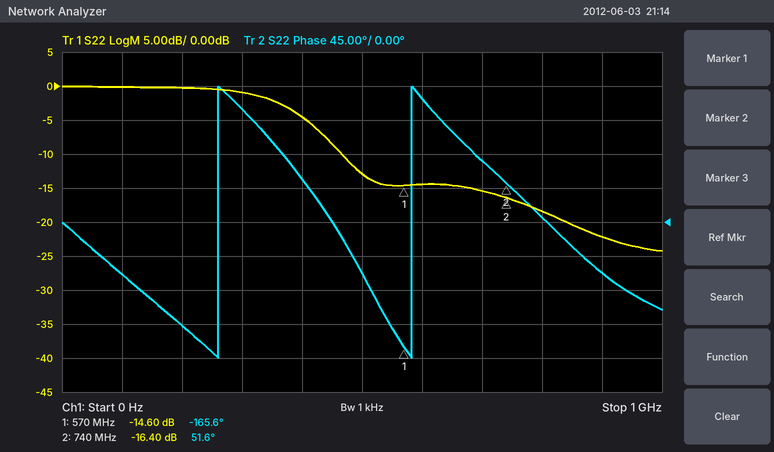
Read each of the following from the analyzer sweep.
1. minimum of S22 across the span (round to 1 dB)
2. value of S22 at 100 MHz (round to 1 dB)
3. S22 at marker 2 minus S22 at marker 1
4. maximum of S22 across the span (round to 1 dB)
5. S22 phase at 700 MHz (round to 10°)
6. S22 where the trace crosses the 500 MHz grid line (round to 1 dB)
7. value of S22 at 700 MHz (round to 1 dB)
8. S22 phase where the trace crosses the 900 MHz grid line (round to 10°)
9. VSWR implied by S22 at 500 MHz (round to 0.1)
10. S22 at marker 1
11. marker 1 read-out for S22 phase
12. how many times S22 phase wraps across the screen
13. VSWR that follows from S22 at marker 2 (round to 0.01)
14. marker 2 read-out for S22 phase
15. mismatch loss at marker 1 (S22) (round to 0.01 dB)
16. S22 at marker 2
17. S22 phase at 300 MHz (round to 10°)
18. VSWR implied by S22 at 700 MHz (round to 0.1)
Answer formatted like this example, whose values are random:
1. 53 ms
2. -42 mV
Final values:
1. -24 dB
2. 0 dB
3. -1.80 dB
4. 0 dB
5. 80°
6. -13 dB
7. -15 dB
8. -70°
9. 1.6
10. -14.60 dB
11. -165.6°
12. 2
13. 1.36
14. 51.6°
15. 0.15 dB
16. -16.40 dB
17. 150°
18. 1.4
